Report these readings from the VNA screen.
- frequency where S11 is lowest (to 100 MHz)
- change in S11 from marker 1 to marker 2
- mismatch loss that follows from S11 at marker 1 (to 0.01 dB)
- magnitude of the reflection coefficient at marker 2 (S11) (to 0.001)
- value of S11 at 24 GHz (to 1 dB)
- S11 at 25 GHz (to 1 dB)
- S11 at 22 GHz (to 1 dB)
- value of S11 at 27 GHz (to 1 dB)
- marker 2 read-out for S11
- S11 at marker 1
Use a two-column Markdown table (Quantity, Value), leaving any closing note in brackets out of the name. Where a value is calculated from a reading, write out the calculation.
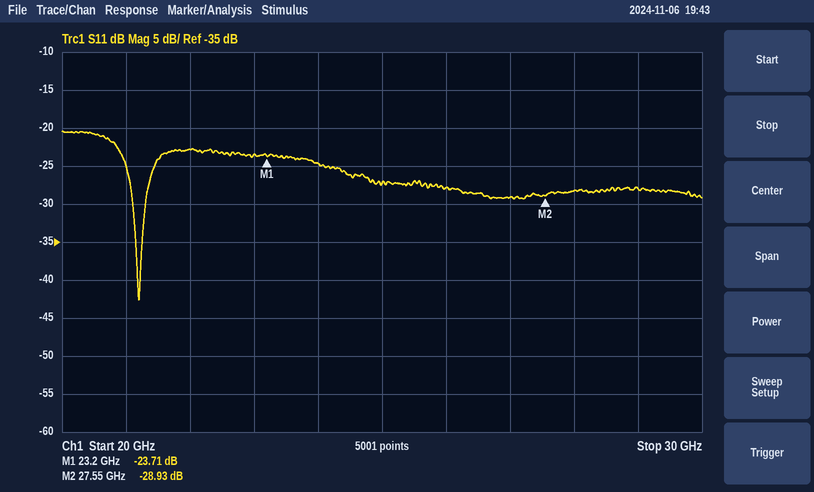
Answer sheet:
| Quantity | Value |
|---|---|
| frequency where S11 is lowest | 21.2 GHz |
| change in S11 from marker 1 to marker 2 | -28.93 − (-23.71) = -5.22 dB |
| mismatch loss that follows from S11 at marker 1 | −10 log10(1 − 10^(-23.71/10)) ≈ 0.02 dB |
| magnitude of the reflection coefficient at marker 2 (S11) | 10^(-28.93/20) ≈ 0.036 |
| value of S11 at 24 GHz | -25 dB |
| S11 at 25 GHz | -27 dB |
| S11 at 22 GHz | -23 dB |
| value of S11 at 27 GHz | -29 dB |
| marker 2 read-out for S11 | -28.93 dB |
| S11 at marker 1 | -23.71 dB |
